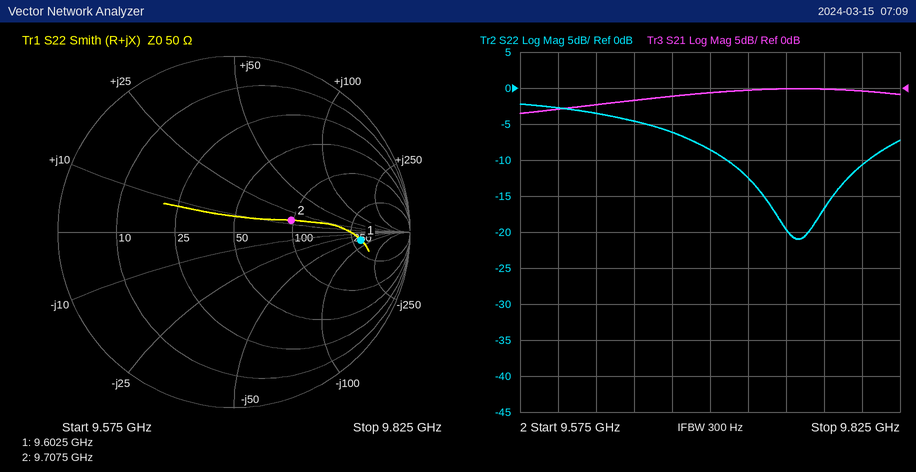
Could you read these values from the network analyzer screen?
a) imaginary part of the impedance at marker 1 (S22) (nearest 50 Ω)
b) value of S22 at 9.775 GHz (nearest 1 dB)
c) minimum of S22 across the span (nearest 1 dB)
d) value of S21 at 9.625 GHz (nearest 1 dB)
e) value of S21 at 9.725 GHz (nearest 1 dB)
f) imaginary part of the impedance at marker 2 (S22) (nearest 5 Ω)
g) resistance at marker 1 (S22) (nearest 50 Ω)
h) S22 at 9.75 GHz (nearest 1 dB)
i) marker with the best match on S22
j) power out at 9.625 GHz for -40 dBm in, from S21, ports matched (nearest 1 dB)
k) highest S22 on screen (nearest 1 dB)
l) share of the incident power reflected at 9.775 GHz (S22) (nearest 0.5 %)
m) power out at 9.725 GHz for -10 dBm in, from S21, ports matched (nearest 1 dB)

-50 Ω
-17 dB
-21 dB
-2 dB
0 dB
+15 Ω
300 Ω
-20 dB
marker 2
-42 dBm
-2 dB
2.0 %
-10 dBm
